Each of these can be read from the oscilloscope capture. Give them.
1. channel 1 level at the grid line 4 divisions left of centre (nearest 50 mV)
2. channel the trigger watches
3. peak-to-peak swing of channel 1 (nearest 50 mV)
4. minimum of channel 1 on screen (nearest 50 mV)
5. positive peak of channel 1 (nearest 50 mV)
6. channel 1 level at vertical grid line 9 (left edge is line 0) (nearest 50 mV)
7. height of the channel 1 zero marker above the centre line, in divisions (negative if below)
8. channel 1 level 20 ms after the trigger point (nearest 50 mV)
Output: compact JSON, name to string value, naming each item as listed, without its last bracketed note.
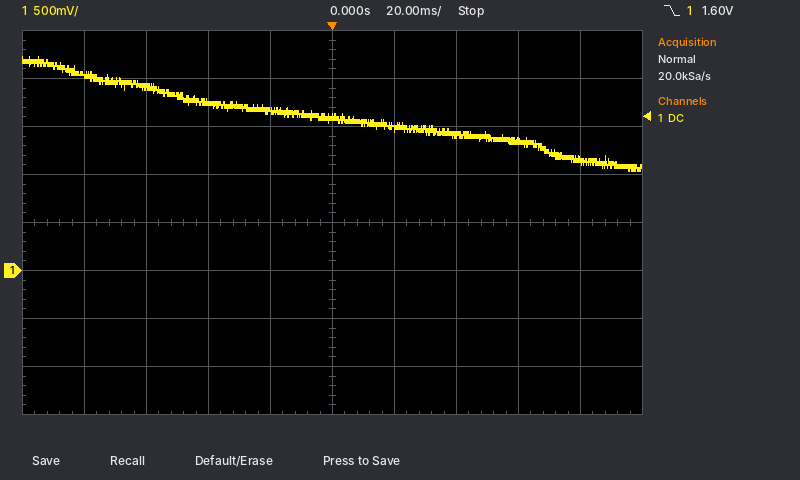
{"channel 1 level at the grid line 4 divisions left of centre": "2.05 V", "channel the trigger watches": "channel 1", "peak-to-peak swing of channel 1": "1.20 V", "minimum of channel 1 on screen": "1.05 V", "positive peak of channel 1": "2.25 V", "channel 1 level at vertical grid line 9 (left edge is line 0)": "1.15 V", "height of the channel 1 zero marker above the centre line, in divisions": "-1.0 div", "channel 1 level 20 ms after the trigger point": "1.50 V"}
